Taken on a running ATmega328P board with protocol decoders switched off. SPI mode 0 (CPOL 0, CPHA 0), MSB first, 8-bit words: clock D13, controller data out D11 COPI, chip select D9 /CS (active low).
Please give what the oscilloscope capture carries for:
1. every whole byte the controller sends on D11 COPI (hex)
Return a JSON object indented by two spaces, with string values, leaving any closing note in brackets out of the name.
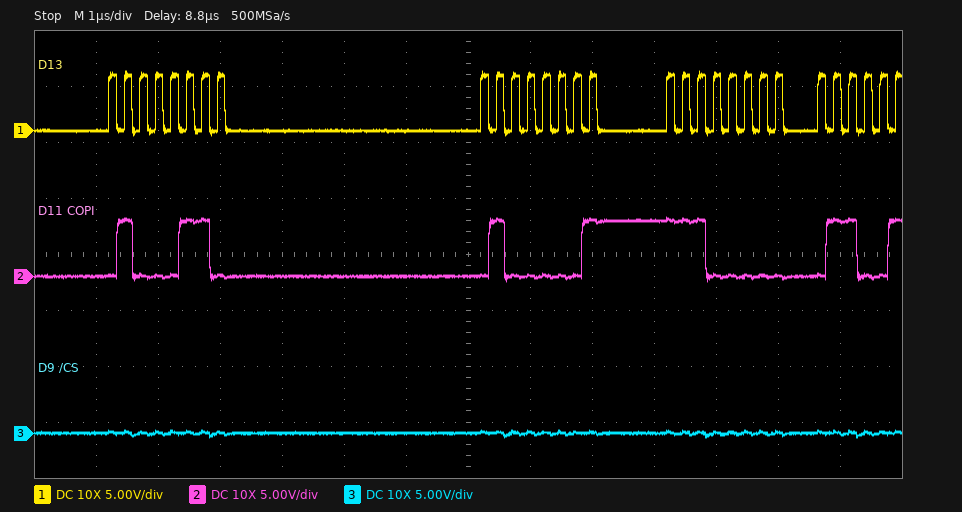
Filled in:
{
  "every whole byte the controller sends on D11 COPI": "46 41 E0"
}
